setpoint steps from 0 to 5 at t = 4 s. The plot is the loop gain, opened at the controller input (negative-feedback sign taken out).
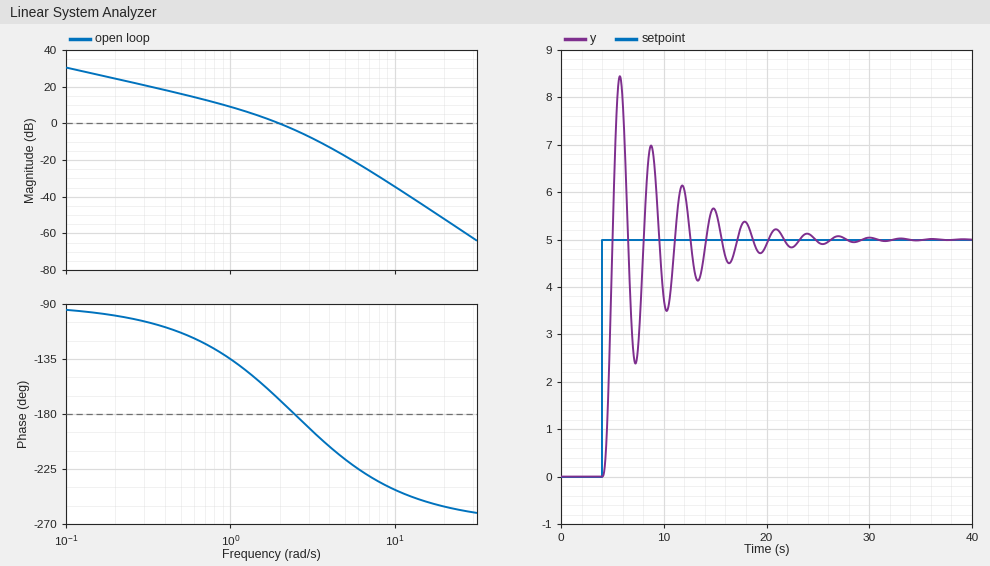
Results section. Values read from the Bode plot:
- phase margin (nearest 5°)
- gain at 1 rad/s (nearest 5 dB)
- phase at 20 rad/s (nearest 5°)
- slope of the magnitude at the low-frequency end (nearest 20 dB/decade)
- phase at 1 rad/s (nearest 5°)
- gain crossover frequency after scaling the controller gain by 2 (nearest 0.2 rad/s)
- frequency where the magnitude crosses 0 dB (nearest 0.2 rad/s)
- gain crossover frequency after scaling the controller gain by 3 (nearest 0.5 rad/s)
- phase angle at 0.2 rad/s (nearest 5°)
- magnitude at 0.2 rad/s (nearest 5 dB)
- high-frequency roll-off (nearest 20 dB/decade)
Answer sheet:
10°
10 dB
-255°
-20 dB/decade
-135°
2.8 rad/s
2.0 rad/s
3.5 rad/s
-100°
25 dB
-60 dB/decade
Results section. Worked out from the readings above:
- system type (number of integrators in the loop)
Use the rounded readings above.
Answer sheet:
1
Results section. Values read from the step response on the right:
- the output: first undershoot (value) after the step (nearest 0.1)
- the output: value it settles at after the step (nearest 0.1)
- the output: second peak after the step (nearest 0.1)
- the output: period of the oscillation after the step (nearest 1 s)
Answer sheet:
2.4
5.0
7.0
3 s
